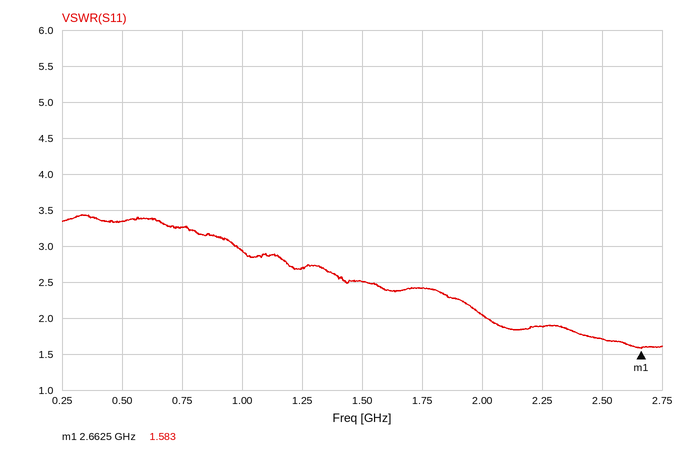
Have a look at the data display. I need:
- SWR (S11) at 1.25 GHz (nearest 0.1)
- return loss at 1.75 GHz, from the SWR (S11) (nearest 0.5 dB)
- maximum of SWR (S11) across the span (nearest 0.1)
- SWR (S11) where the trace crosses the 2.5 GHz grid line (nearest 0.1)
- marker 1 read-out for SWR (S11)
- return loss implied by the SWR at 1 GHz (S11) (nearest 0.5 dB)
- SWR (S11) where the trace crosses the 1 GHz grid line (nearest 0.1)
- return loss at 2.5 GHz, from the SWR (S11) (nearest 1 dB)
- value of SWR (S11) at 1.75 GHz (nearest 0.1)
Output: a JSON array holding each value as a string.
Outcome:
["2.7", "7.5 dB", "3.4", "1.7", "1.583", "6.0 dB", "2.9", "12 dB", "2.4"]
